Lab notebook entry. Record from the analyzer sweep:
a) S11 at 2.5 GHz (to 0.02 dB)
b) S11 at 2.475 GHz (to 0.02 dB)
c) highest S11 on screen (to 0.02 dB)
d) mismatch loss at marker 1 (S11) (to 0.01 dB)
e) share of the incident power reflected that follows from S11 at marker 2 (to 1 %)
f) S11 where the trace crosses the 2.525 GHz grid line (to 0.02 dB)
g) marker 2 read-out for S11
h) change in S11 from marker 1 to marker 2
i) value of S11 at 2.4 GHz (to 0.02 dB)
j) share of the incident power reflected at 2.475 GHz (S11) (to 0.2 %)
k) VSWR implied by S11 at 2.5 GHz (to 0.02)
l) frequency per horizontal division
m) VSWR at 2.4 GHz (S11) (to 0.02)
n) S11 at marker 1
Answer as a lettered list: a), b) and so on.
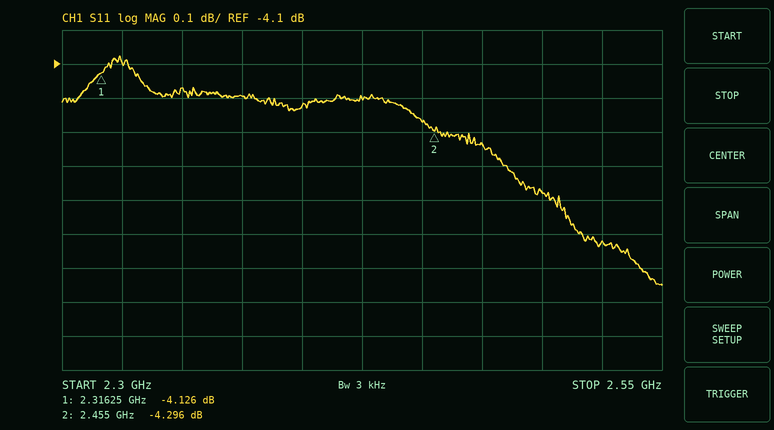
a) -4.48 dB
b) -4.34 dB
c) -4.08 dB
d) 2.12 dB
e) 37 %
f) -4.62 dB
g) -4.296 dB
h) -0.170 dB
i) -4.22 dB
j) 36.8 %
k) 3.96
l) 25 MHz
m) 4.20
n) -4.126 dB
